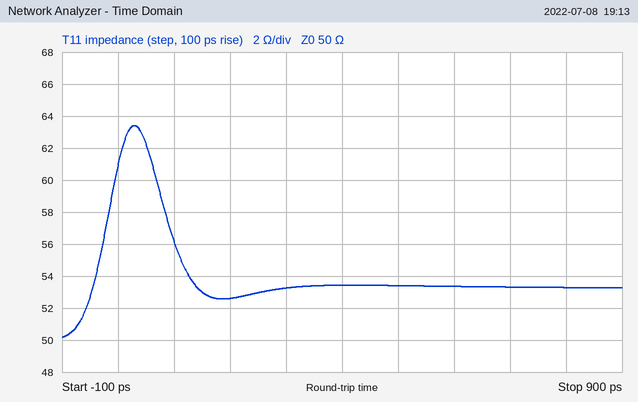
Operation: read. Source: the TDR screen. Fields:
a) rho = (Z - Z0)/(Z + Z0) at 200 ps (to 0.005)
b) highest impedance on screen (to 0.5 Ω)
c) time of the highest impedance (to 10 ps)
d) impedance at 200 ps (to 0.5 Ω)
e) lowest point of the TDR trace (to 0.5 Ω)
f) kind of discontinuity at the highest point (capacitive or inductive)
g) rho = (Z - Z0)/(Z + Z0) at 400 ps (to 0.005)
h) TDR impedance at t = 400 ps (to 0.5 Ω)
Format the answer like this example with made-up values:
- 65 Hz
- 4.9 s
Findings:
- +0.025
- 63.5 Ω
- 30 ps
- 52.5 Ω
- 50.0 Ω
- inductive
- +0.035
- 53.5 Ω
